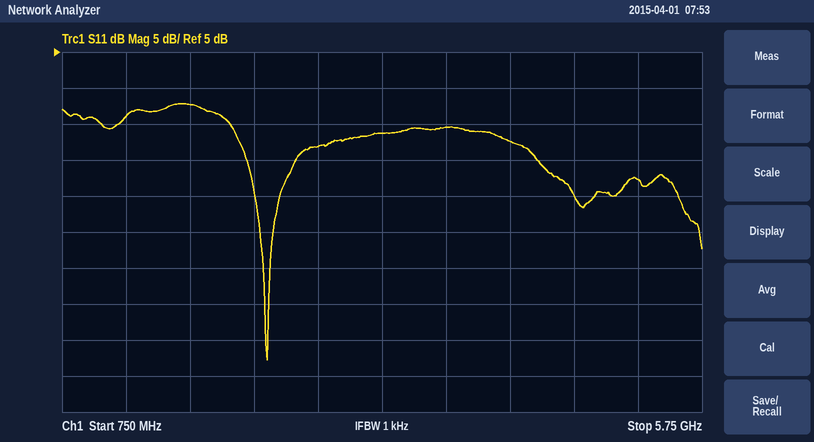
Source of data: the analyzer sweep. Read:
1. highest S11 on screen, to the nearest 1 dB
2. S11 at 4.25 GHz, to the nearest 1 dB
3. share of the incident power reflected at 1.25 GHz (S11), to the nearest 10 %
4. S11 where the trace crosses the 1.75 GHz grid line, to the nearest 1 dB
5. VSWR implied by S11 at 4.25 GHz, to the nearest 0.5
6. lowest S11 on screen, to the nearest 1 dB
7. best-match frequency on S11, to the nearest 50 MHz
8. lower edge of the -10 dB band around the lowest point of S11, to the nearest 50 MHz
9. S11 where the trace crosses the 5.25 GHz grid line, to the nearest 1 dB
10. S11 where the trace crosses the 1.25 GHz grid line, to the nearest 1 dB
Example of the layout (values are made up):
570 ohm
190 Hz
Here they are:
-2 dB
-7 dB
40 %
-2 dB
2.5
-38 dB
2.35 GHz
2.20 GHz
-13 dB
-4 dB
